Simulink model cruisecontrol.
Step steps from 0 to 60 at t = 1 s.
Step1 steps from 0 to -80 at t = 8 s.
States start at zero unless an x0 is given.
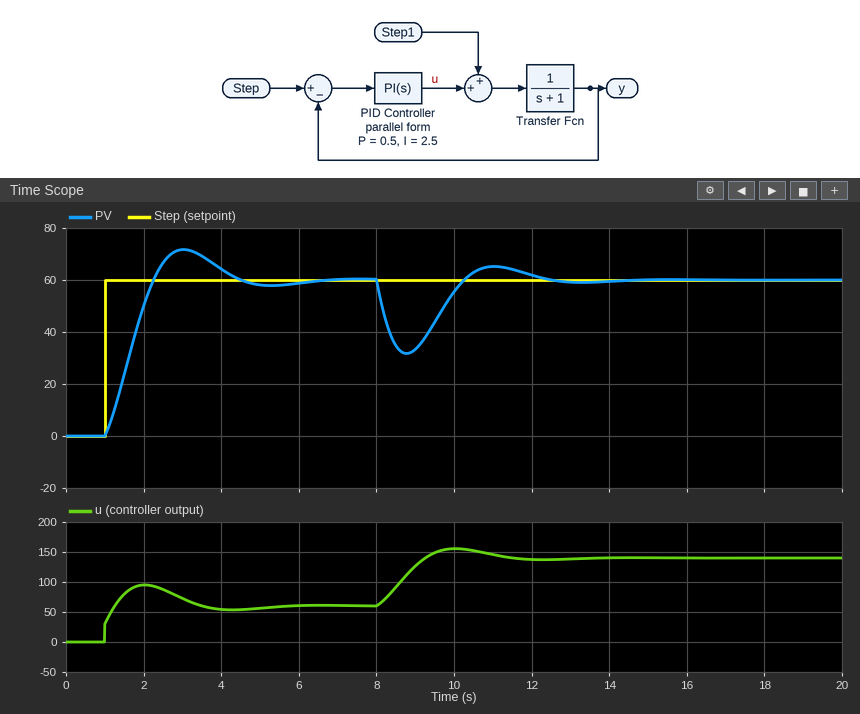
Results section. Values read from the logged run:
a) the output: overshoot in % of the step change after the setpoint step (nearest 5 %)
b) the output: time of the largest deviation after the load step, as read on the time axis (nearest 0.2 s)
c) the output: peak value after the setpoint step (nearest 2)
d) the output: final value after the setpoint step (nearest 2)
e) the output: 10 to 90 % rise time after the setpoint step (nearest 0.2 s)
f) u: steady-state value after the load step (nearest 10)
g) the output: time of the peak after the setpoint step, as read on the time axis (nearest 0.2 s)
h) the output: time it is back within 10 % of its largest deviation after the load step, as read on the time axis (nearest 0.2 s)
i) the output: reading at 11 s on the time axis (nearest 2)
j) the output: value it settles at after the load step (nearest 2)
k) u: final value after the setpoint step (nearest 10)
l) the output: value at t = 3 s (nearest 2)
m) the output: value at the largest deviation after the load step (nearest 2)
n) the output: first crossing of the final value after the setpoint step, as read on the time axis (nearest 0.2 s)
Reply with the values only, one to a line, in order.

20 %
8.8 s
72
60
1.0 s
140
3.0 s
11.8 s
66
60
60
72
32
2.2 s
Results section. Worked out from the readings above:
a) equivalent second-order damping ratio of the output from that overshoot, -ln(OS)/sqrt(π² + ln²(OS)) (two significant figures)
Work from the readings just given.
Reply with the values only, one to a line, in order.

0.46
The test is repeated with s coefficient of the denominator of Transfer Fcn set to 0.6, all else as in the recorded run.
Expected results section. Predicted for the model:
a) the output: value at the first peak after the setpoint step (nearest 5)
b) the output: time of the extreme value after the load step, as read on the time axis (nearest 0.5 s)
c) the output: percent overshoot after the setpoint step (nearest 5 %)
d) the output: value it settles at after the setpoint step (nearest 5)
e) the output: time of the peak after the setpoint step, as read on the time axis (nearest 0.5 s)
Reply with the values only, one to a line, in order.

65
8.5 s
10 %
60
2.5 s
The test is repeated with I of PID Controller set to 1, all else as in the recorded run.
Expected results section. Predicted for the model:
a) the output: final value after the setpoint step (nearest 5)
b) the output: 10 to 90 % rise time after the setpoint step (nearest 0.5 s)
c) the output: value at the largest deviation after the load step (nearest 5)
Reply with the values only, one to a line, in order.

60
2.0 s
25
